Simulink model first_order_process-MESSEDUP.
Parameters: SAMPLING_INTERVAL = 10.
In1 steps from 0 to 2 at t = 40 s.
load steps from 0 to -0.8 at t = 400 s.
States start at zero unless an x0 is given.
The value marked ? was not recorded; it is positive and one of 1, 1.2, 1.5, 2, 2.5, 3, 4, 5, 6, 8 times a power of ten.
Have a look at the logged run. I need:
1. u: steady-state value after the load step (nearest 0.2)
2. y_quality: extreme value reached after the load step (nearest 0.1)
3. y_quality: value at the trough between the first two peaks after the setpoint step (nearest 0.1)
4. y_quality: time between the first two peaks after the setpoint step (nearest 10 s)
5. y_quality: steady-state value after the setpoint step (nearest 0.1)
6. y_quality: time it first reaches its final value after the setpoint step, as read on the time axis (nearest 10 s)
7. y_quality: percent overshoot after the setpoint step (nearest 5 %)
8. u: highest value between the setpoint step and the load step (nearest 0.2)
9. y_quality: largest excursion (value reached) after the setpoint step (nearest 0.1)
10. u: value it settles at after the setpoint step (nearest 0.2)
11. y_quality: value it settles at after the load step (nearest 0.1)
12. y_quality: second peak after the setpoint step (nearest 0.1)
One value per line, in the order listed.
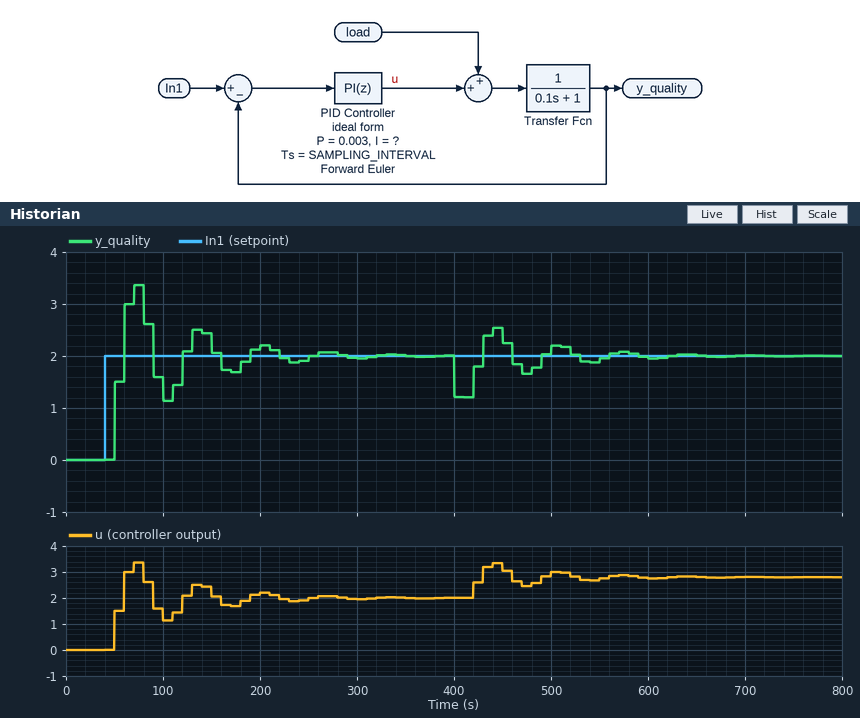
2.8
1.2
1.1
60 s
2.0
60 s
70 %
3.4
3.4
2.0
2.0
2.5
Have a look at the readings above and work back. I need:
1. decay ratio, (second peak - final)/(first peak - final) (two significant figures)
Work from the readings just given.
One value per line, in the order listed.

0.36
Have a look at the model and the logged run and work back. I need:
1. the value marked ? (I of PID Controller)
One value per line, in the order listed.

25
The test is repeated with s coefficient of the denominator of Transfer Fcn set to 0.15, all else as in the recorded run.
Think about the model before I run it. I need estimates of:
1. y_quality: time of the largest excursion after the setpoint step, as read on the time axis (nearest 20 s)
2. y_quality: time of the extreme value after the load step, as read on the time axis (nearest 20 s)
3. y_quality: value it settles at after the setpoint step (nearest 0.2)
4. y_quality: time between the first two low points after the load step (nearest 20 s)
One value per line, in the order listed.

80 s
420 s
2.0
60 s
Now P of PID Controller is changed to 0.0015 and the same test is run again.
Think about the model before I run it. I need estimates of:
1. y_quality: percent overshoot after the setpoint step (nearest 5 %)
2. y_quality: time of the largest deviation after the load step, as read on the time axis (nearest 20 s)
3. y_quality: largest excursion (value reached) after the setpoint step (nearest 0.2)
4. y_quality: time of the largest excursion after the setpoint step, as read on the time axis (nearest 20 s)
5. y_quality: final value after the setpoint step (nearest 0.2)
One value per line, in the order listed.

10 %
400 s
2.2
100 s
2.0
